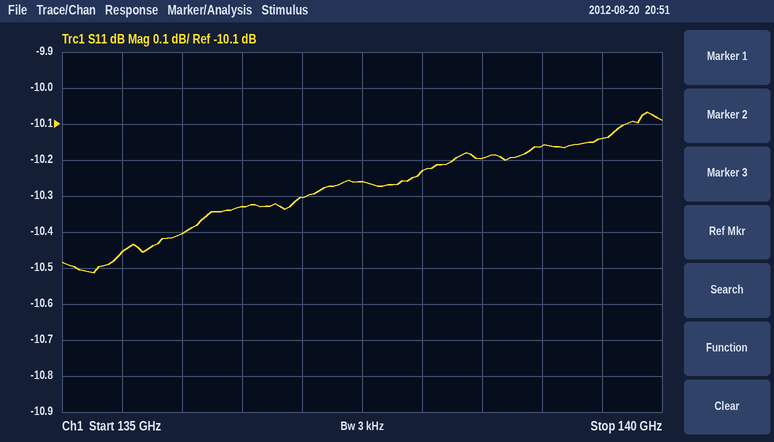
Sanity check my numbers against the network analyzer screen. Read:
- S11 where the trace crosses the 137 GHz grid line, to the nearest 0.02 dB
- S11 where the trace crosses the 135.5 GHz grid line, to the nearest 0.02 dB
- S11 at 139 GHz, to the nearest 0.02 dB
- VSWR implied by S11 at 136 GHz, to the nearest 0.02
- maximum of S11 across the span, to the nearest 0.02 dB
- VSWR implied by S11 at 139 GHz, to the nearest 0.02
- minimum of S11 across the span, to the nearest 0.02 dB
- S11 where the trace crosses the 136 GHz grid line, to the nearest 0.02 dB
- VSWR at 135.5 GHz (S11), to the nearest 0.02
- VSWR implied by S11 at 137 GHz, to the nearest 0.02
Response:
-10.30 dB
-10.46 dB
-10.16 dB
1.86
-10.06 dB
1.90
-10.52 dB
-10.40 dB
1.86
1.88
